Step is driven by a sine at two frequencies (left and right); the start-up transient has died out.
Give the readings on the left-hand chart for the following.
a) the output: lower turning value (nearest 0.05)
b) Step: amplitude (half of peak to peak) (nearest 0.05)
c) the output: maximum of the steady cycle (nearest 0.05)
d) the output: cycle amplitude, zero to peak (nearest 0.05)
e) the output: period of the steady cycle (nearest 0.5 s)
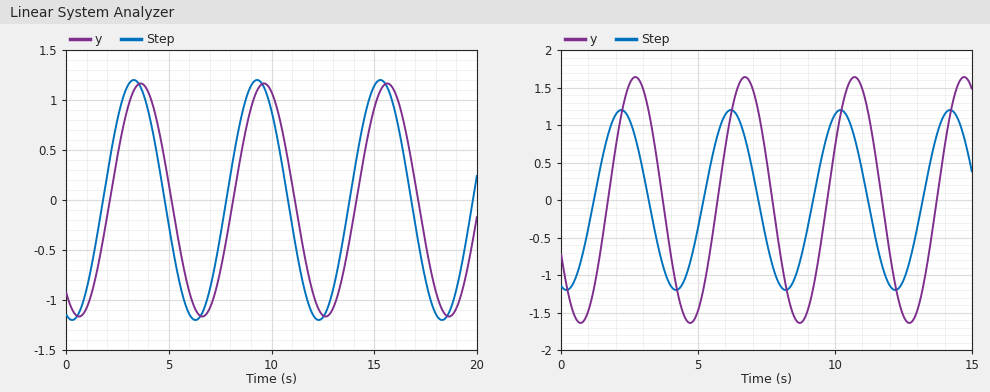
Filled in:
-1.15
1.20
1.15
1.15
6.0 s
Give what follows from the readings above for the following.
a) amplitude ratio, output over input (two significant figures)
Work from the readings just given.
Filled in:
0.96
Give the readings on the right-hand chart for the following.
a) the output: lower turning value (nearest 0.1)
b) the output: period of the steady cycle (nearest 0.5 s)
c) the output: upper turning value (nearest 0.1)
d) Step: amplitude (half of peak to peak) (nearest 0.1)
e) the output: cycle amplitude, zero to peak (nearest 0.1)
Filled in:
-1.6
4.0 s
1.6
1.2
1.6
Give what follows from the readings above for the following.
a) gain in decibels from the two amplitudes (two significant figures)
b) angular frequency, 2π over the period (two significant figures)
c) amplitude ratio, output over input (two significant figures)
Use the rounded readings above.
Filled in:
2.5 dB
1.6 rad/s
1.3
